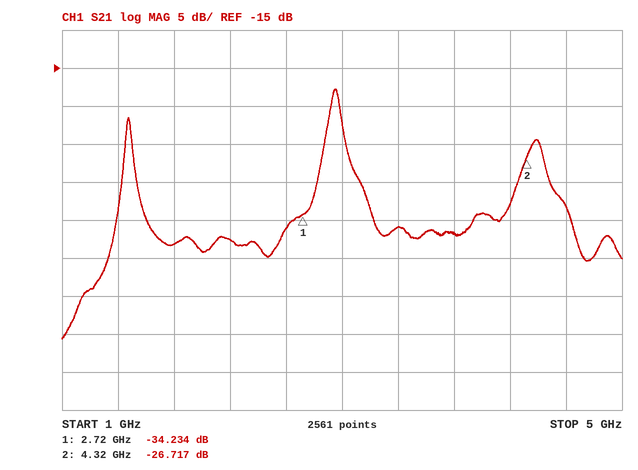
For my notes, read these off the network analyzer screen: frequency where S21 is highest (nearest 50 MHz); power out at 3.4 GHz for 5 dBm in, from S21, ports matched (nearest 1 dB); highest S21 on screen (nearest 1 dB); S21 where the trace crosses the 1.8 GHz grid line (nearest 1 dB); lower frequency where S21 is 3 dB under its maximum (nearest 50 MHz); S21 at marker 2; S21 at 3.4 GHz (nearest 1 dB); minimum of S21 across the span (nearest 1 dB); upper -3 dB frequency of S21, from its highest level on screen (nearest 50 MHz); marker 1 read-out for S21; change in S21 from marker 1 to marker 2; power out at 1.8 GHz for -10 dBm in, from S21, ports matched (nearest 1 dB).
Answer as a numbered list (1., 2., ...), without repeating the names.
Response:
1. 2.95 GHz
2. -31 dBm
3. -18 dB
4. -38 dB
5. 2.90 GHz
6. -26.717 dB
7. -36 dB
8. -51 dB
9. 3.00 GHz
10. -34.234 dB
11. 7.517 dB
12. -48 dBm
